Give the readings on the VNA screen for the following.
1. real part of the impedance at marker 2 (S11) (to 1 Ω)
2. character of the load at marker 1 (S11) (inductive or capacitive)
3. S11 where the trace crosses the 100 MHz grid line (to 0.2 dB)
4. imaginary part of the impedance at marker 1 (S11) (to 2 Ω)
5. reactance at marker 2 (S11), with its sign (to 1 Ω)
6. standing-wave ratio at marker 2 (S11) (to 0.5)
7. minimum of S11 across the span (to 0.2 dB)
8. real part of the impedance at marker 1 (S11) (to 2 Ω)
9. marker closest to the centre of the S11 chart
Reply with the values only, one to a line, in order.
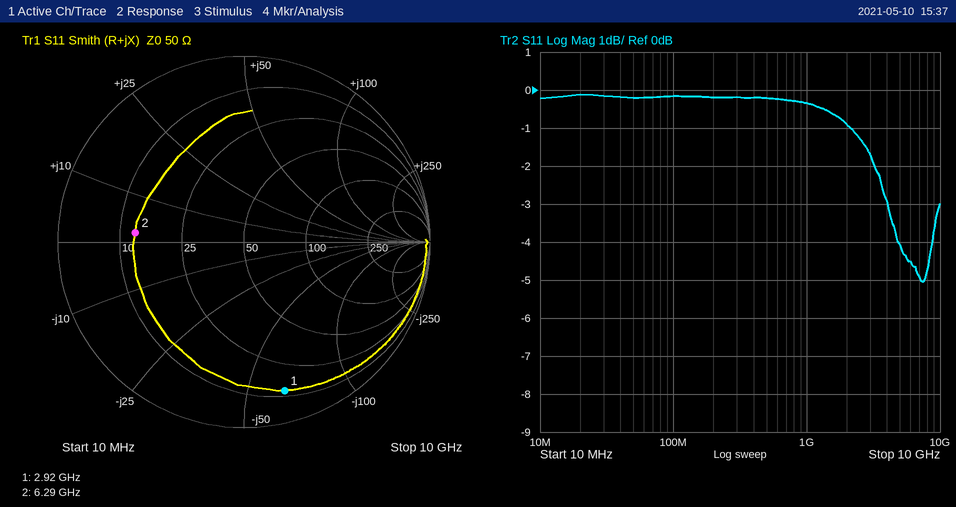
13 Ω
capacitive
-0.2 dB
-64 Ω
+2 Ω
4.0
-5.0 dB
12 Ω
marker 2
